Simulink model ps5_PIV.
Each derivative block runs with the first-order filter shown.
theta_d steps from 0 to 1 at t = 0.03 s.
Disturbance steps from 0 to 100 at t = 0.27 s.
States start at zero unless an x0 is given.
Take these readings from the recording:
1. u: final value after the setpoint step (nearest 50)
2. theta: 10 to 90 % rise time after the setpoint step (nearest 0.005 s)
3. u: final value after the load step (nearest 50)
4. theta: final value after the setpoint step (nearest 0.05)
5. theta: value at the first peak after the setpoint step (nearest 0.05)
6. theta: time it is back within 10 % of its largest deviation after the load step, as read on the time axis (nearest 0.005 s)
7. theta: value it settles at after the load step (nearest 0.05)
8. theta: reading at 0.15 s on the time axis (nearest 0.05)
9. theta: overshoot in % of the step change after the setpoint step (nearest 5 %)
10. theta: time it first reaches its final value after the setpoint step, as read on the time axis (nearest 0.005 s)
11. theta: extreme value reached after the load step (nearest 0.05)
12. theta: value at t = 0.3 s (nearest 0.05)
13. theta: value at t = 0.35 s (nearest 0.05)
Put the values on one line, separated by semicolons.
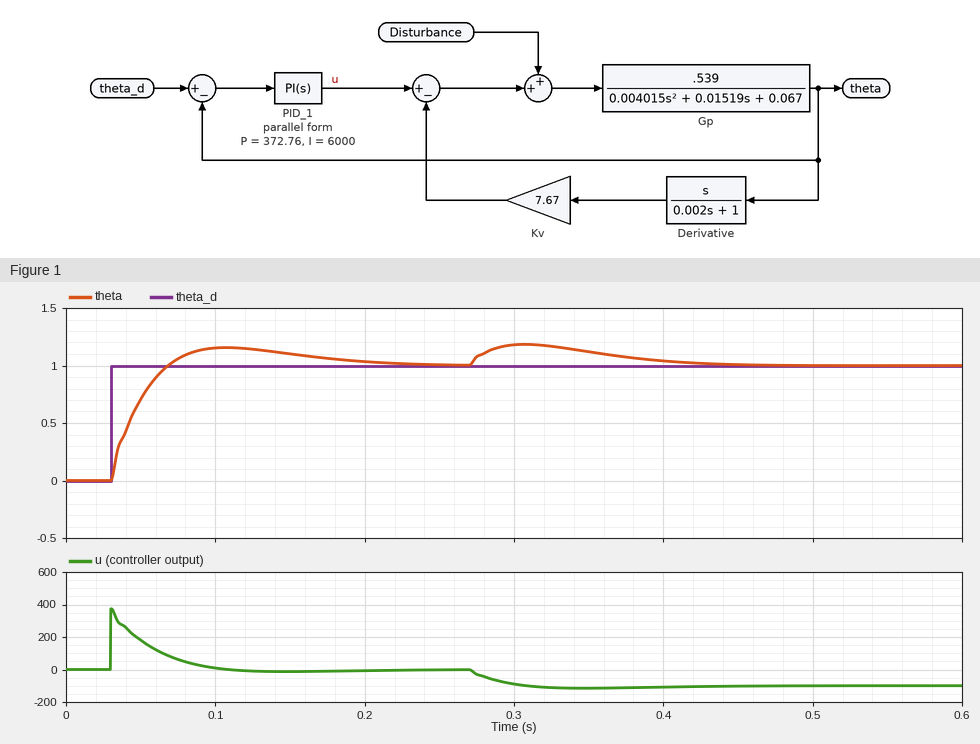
0; 0.030 s; -100; 1.00; 1.15; 0.425 s; 1.00; 1.10; 15 %; 0.070 s; 1.20; 1.20; 1.10
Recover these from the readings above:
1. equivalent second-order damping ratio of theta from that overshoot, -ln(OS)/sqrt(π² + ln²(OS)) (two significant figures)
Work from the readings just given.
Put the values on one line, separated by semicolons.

0.52
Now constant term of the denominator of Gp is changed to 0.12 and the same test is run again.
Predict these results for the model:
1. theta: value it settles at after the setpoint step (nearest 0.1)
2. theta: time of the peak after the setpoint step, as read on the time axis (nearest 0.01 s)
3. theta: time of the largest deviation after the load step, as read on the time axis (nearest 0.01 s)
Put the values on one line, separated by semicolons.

1.0; 0.11 s; 0.31 s
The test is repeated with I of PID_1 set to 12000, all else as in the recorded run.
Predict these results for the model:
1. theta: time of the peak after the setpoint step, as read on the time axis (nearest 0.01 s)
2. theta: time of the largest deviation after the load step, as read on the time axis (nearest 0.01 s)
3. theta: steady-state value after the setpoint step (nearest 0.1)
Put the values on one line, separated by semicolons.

0.09 s; 0.30 s; 1.0
